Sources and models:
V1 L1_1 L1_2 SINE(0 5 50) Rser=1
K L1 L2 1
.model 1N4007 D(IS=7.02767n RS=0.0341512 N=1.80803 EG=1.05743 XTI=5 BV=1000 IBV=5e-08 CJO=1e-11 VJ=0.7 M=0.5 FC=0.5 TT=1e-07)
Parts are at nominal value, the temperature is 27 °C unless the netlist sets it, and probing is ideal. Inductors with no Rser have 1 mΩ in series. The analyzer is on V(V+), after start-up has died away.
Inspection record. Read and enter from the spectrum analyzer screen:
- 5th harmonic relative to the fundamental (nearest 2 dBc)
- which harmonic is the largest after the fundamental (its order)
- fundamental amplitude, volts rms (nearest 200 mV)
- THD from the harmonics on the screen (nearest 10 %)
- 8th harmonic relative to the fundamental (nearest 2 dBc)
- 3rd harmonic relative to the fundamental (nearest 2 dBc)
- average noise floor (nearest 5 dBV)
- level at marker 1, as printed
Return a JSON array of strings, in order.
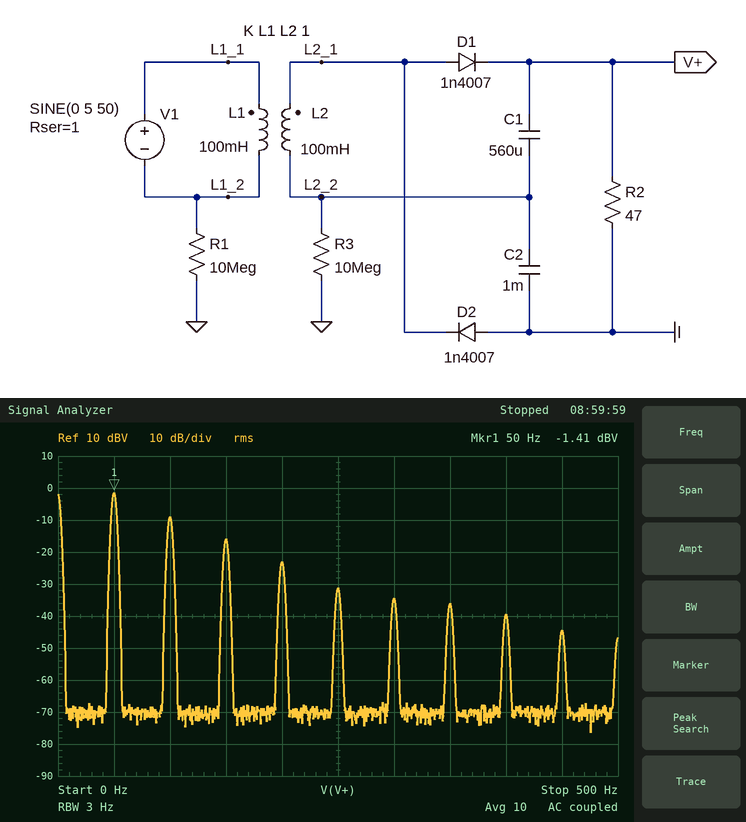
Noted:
["-30 dBc", "2", "800 mV", "50 %", "-38 dBc", "-14 dBc", "-70 dBV", "-1.41 dBV"]
